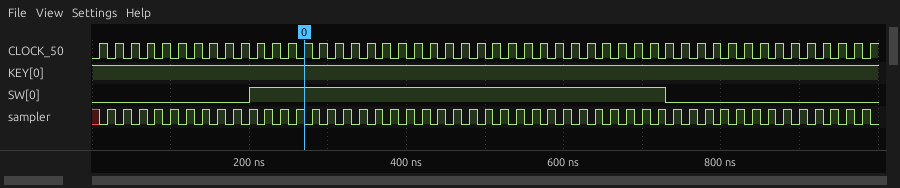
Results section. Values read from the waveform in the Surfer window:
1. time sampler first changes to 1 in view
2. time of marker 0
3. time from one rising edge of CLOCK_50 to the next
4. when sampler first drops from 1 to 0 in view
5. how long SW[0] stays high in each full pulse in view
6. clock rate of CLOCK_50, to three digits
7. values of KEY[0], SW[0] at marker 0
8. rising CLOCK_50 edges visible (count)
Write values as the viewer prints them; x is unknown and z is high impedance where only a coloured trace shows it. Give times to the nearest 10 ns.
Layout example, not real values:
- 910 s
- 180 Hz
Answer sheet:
- 20 ns
- 270 ns
- 20 ns
- 30 ns
- 530 ns
- 50.0 MHz
- KEY[0]=1, SW[0]=1
- 50
